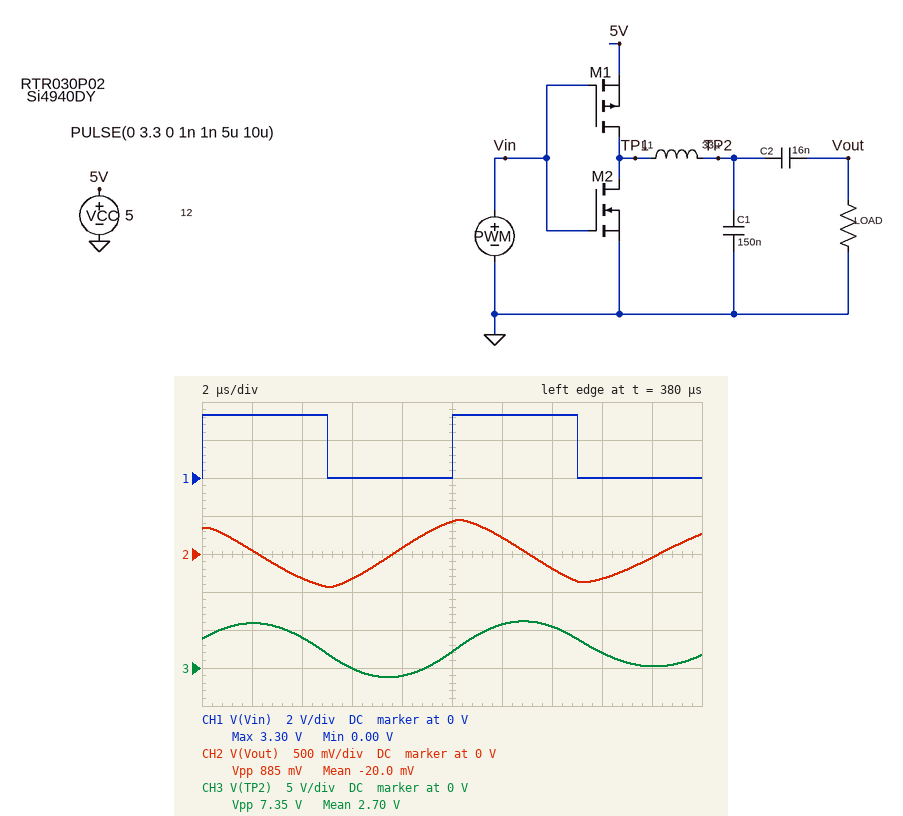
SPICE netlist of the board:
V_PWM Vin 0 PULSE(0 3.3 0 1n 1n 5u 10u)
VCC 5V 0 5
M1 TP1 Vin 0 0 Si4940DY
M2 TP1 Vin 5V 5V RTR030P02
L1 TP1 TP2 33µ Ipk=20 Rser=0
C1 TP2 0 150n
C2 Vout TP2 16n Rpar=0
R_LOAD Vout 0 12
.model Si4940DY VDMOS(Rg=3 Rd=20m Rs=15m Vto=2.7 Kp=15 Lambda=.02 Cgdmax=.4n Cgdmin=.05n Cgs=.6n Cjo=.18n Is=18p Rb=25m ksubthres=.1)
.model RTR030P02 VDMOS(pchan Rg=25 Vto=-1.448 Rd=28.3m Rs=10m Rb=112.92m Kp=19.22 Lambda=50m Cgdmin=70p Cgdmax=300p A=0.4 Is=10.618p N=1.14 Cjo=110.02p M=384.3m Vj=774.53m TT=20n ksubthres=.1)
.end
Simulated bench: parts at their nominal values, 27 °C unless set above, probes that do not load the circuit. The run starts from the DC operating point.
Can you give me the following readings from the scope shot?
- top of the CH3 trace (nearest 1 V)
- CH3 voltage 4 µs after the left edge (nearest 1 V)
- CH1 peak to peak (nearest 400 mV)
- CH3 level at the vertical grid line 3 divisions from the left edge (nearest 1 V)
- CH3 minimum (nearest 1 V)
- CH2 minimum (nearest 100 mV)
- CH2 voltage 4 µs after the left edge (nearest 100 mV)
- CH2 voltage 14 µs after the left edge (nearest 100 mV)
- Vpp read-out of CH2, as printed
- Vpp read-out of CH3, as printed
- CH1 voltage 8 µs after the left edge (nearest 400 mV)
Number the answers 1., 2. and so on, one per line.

1. 6 V
2. 4 V
3. 3.2 V
4. 0 V
5. -1 V
6. -400 mV
7. -300 mV
8. -200 mV
9. 885 mV
10. 7.35 V
11. 0 V
